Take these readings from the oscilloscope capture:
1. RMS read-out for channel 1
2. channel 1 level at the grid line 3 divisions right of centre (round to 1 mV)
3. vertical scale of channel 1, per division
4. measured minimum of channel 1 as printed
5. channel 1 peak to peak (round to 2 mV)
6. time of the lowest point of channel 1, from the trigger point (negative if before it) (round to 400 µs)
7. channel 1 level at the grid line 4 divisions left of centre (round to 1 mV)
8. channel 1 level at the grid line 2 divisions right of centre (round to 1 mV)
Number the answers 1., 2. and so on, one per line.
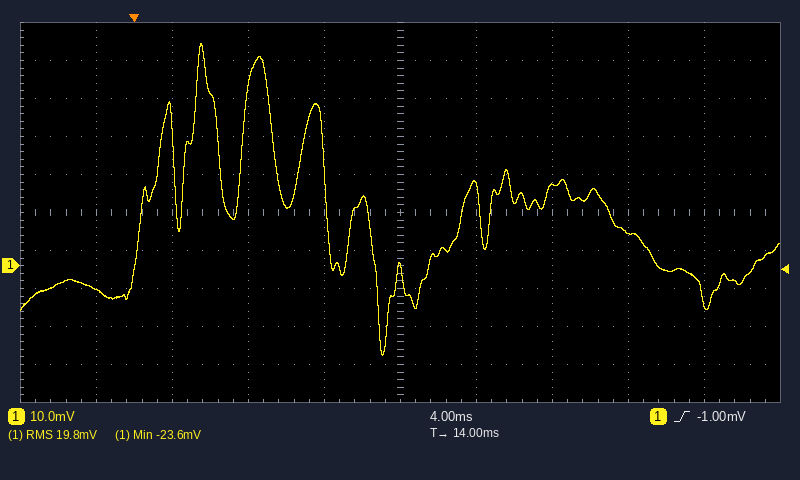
1. 19.8 mV
2. 9 mV
3. 10 mV
4. -23.6 mV
5. 82 mV
6. +13.2 ms
7. -6 mV
8. 21 mV
